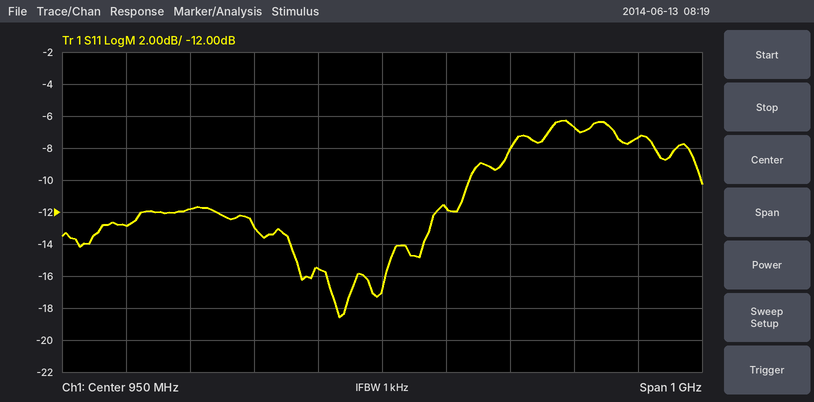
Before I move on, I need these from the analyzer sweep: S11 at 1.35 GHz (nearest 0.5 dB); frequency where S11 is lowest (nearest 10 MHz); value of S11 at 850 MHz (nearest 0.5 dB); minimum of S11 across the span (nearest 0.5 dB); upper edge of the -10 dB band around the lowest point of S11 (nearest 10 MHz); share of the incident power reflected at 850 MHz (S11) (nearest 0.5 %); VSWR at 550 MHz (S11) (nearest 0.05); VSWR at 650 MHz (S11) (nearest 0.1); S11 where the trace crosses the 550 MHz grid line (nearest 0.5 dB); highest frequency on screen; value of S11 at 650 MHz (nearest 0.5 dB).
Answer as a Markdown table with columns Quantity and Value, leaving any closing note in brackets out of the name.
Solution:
| Quantity | Value |
|---|---|
| S11 at 1.35 GHz | -7.5 dB |
| frequency where S11 is lowest | 880 MHz |
| value of S11 at 850 MHz | -15.5 dB |
| minimum of S11 across the span | -18.5 dB |
| upper edge of the -10 dB band around the lowest point of S11 | 1.09 GHz |
| share of the incident power reflected at 850 MHz (S11) | 3.0 % |
| VSWR at 550 MHz (S11) | 1.60 |
| VSWR at 650 MHz (S11) | 1.7 |
| S11 where the trace crosses the 550 MHz grid line | -13.0 dB |
| highest frequency on screen | 1.45 GHz |
| value of S11 at 650 MHz | -12.0 dB |
